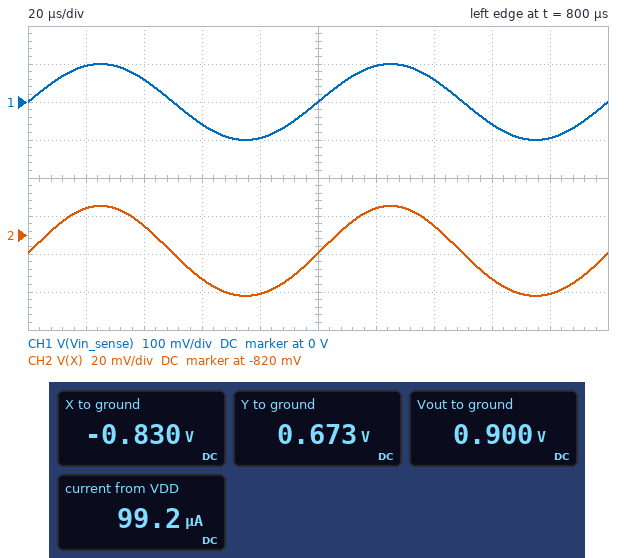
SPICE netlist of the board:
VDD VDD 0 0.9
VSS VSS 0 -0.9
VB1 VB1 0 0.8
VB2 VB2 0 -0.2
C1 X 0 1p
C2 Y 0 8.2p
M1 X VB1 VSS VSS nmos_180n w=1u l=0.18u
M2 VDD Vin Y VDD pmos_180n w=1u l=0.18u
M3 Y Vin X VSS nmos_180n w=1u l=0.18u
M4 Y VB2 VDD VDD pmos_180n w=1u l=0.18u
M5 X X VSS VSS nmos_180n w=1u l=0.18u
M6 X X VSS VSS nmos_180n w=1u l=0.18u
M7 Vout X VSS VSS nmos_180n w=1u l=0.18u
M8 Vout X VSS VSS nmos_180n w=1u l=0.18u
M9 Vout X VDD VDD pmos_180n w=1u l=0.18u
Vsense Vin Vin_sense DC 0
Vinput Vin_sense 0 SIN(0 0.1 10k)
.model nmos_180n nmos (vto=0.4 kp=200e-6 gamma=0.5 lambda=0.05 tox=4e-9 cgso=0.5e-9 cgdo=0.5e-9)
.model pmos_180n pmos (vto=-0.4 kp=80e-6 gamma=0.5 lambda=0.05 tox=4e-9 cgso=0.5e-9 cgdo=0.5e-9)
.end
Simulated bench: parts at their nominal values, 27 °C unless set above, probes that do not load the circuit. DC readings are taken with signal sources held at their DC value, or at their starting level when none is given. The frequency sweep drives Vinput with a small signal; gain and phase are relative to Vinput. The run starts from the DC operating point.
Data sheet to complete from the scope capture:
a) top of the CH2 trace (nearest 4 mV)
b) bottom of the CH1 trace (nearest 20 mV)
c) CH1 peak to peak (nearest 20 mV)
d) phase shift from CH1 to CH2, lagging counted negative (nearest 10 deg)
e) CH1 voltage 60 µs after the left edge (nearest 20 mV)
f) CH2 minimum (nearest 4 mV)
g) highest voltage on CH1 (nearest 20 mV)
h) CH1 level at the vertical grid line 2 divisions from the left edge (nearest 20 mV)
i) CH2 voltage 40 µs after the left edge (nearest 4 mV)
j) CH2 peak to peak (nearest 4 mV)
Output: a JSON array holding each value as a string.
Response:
["-804 mV", "-100 mV", "200 mV", "0 deg", "-60 mV", "-852 mV", "100 mV", "60 mV", "-816 mV", "48 mV"]
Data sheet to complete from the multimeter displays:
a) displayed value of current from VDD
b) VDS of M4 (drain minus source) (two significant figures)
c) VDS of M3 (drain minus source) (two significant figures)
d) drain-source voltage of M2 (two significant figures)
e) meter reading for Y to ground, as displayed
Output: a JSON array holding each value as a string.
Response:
["99.2 µA", "-230 mV", "1.5 V", "230 mV", "0.673 V"]
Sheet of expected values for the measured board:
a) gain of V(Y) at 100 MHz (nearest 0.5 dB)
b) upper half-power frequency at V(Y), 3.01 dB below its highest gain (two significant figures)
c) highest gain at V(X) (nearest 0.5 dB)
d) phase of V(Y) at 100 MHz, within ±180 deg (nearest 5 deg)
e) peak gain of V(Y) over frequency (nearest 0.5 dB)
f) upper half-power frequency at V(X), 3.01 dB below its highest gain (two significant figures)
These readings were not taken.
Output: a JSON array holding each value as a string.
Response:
["-21.0 dB", "6.7 MHz", "-12.5 dB", "100 deg", "2.0 dB", "320 MHz"]
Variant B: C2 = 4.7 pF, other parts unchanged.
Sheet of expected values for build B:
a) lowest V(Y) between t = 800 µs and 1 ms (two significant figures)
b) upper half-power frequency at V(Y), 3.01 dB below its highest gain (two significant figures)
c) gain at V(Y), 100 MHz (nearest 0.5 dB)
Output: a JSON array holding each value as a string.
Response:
["450 mV", "12 MHz", "-16.5 dB"]
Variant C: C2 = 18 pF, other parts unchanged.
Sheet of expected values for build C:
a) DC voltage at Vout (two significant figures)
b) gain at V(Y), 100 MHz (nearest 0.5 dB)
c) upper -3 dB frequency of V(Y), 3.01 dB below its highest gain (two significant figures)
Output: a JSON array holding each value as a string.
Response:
["900 mV", "-28.0 dB", "3.0 MHz"]
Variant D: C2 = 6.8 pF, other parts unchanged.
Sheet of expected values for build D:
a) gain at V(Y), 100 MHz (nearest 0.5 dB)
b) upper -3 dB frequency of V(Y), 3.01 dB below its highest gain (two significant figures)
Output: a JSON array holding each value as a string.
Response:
["-19.5 dB", "8.0 MHz"]
